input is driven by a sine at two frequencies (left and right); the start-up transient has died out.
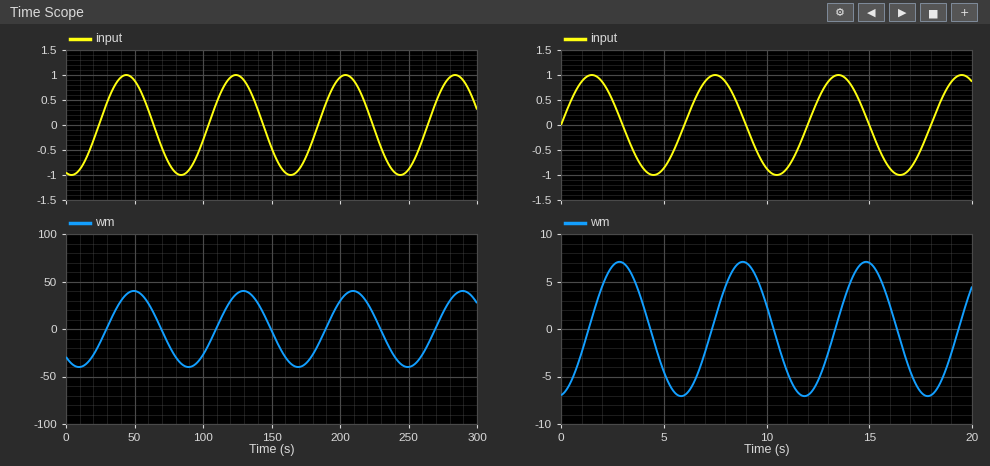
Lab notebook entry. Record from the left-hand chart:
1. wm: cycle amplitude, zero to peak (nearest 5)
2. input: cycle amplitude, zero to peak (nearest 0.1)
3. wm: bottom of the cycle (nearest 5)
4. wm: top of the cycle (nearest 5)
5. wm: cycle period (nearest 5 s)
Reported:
40
1.0
-40
40
80 s
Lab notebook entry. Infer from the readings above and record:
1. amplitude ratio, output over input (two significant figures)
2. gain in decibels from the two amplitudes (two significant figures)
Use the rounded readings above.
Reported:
40
32 dB
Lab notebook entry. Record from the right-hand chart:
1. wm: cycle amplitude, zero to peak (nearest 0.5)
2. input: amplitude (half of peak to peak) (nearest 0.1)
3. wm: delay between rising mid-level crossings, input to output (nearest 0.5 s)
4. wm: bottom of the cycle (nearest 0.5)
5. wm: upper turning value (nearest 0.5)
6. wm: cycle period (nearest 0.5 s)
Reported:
7.0
1.0
1.5 s
-7.0
7.0
6.0 s
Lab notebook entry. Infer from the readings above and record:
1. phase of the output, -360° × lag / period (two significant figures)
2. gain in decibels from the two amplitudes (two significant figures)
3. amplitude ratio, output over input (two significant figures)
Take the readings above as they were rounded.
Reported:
-90°
17 dB
7.0
